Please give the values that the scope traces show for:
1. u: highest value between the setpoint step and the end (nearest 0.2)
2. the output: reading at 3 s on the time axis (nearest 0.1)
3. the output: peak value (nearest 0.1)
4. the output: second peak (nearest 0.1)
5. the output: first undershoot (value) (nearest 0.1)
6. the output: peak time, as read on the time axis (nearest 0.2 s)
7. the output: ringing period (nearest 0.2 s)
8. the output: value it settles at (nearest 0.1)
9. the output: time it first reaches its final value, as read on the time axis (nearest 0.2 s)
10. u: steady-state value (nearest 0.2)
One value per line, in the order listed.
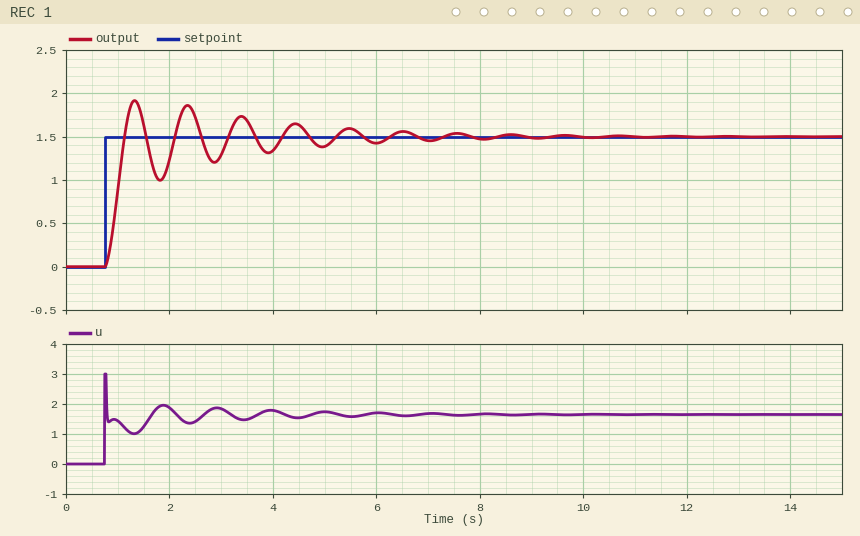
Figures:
3.0
1.3
1.9
1.9
1.0
1.4 s
1.0 s
1.5
1.2 s
1.6
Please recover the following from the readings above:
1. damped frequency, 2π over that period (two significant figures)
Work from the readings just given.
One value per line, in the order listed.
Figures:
6.3 rad/s
